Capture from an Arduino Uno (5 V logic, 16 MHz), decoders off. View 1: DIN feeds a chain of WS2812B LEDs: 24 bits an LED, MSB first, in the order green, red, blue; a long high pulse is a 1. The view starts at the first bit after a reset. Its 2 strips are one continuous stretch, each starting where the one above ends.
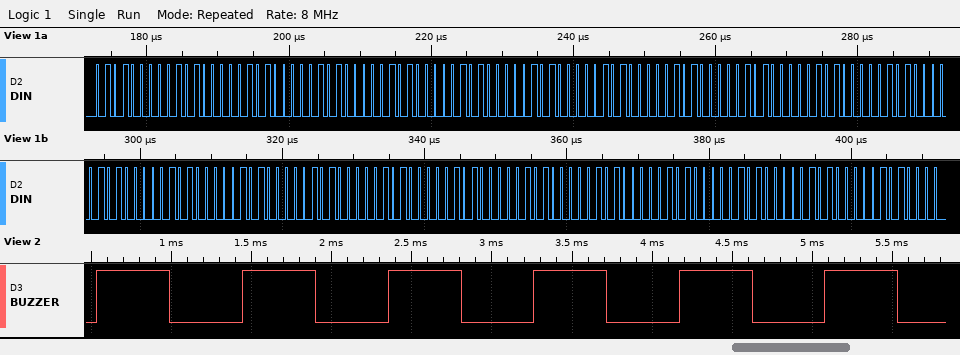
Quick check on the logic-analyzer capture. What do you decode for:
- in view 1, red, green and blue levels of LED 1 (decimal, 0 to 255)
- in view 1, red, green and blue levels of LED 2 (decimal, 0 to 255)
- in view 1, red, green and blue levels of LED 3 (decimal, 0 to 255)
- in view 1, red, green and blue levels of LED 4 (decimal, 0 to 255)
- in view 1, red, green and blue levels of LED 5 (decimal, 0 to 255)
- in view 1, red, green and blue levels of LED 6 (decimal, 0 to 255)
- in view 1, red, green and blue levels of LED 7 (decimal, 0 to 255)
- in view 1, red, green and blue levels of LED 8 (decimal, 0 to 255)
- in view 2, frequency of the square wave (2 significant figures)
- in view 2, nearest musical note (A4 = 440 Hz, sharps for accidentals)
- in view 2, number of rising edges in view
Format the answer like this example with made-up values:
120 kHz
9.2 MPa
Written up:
80, 80, 80
80, 80, 80
80, 80, 80
80, 80, 80
80, 80, 80
80, 80, 80
80, 80, 80
80, 80, 80
1.1 kHz
C#6
6
